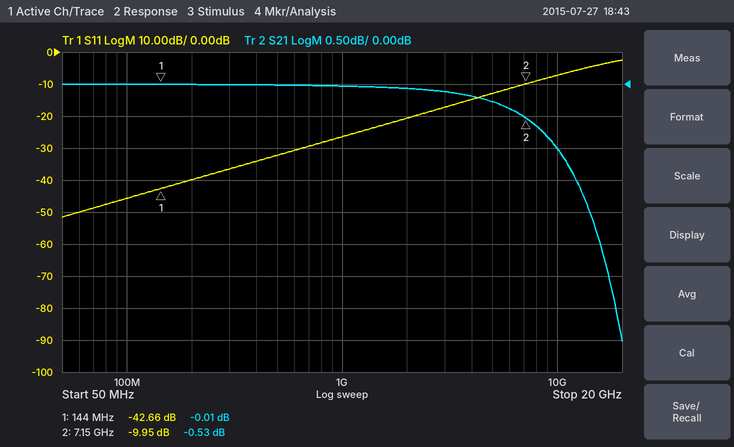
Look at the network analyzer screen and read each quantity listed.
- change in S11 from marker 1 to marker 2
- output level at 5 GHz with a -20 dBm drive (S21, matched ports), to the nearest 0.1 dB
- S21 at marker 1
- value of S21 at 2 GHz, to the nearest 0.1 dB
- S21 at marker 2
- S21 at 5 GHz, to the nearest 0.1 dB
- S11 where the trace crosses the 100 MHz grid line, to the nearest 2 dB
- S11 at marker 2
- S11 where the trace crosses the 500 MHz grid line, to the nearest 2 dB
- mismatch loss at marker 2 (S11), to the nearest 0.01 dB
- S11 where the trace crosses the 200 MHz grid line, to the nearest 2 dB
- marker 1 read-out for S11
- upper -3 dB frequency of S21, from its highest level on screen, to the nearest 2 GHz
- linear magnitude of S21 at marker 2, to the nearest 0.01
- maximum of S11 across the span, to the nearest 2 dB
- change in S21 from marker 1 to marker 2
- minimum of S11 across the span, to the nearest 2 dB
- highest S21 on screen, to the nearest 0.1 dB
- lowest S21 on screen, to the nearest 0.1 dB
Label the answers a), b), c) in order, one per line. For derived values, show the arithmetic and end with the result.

a) -9.95 − (-42.66) = 32.71 dB
b) -20 dBm + (-0.3 dB) = -20.3 dBm
c) -0.01 dB
d) -0.1 dB
e) -0.53 dB
f) -0.3 dB
g) -46 dB
h) -9.95 dB
i) -32 dB
j) −10 log10(1 − 10^(-9.95/10)) ≈ 0.46 dB
k) -40 dB
l) -42.66 dB
m) 18 GHz
n) 10^(-0.53/20) ≈ 0.94
o) -2 dB
p) -0.53 − (-0.01) = -0.52 dB
q) -52 dB
r) 0.0 dB
s) -4.0 dB
